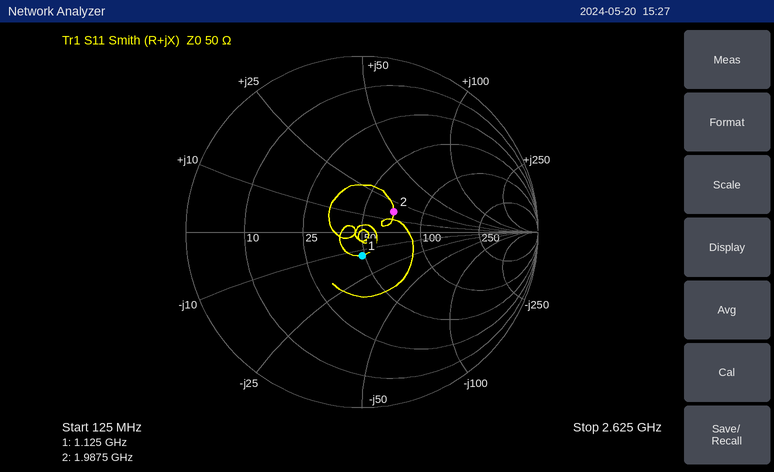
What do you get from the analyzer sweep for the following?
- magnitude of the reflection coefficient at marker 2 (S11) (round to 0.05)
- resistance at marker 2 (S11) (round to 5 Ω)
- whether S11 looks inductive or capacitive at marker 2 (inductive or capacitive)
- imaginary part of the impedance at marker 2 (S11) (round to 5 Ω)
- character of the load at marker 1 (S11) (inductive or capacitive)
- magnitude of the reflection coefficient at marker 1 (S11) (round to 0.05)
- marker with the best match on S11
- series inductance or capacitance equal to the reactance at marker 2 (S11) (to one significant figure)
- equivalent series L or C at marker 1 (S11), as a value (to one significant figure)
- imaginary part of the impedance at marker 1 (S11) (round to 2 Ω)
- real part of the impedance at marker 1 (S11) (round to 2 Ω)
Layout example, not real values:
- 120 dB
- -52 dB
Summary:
- 0.20
- 70 Ω
- inductive
- +15 Ω
- capacitive
- 0.15
- marker 1
- 1 nH
- 10 pF
- -14 Ω
- 48 Ω
